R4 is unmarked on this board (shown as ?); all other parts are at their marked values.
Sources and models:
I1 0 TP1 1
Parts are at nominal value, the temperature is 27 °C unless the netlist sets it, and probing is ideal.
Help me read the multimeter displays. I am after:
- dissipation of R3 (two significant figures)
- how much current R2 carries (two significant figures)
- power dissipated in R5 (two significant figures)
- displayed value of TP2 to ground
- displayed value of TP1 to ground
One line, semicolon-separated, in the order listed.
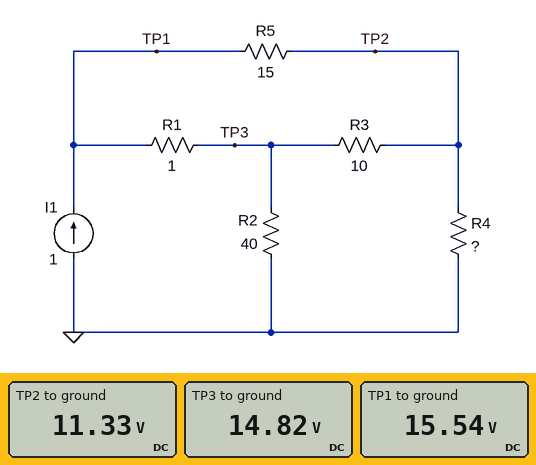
1.2 W; 370 mA; 1.2 W; 11.33 V; 15.54 V
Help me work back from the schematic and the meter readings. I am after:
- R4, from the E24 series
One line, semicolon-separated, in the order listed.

18 Ω
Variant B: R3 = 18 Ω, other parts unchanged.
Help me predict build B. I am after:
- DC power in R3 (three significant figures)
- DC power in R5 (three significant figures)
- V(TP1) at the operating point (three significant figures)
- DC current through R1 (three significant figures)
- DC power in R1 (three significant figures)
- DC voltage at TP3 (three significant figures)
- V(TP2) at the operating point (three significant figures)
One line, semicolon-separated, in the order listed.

1.19 W; 1.86 W; 16.3 V; 648 mA; 420 mW; 15.6 V; 11.0 V
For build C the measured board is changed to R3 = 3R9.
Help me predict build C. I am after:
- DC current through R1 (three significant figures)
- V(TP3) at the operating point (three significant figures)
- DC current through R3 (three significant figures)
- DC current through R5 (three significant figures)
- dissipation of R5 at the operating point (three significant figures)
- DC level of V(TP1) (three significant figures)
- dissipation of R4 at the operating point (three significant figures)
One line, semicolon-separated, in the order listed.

821 mA; 13.7 V; 478 mA; 179 mA; 481 mW; 14.5 V; 7.78 W
